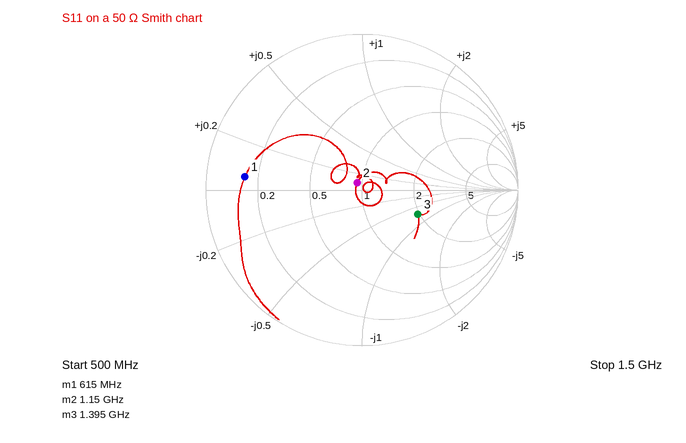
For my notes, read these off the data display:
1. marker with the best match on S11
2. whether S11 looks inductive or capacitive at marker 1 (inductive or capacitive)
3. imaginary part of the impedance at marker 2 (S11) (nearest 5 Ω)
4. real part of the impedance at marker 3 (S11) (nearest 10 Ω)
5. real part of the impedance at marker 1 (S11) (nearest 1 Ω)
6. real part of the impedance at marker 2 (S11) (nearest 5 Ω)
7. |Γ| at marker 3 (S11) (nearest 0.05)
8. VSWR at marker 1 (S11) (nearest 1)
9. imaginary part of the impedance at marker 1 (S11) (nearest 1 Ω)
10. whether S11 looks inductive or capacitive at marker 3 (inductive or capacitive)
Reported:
marker 2
inductive
+5 Ω
100 Ω
7 Ω
45 Ω
0.40
7
+3 Ω
capacitive
